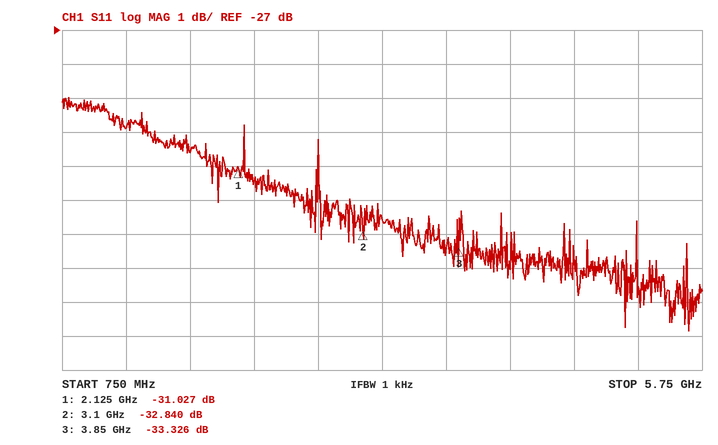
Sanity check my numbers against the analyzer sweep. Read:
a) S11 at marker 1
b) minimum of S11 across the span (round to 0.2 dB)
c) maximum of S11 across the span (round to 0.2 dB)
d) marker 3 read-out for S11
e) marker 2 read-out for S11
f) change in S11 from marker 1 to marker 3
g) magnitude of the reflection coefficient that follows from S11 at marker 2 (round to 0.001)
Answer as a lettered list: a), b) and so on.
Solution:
a) -31.027 dB
b) -35.8 dB
c) -29.0 dB
d) -33.326 dB
e) -32.840 dB
f) -2.299 dB
g) 0.023
